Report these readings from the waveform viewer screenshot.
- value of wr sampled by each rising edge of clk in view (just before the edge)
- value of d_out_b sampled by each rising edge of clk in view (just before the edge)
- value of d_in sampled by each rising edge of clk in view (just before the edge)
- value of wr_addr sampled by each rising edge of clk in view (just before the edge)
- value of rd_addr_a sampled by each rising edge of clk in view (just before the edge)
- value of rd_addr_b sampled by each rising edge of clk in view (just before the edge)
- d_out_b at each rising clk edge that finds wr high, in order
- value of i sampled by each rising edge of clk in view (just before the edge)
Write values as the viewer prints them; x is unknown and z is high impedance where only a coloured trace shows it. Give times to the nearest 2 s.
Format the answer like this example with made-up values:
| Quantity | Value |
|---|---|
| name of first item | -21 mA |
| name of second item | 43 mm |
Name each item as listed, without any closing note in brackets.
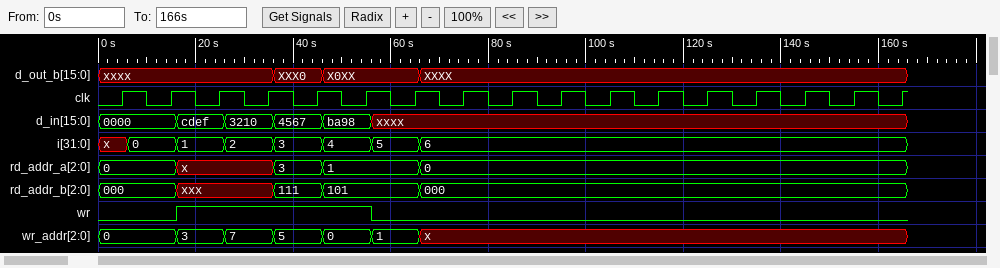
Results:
| Quantity | Value |
|---|---|
| value of wr sampled by each rising edge of clk in view | 0 0 1 1 1 1 0 0 0 0 0 0 0 0 0 0 0 |
| value of d_out_b sampled by each rising edge of clk in view | xxxx, xxxx, xxxx, xxxx, XXX0, X0XX, X0XX, XXXX, XXXX, XXXX, XXXX, XXXX, XXXX, XXXX, XXXX, XXXX, XXXX |
| value of d_in sampled by each rising edge of clk in view | 0000, 0000, cdef, 3210, 4567, ba98, xxxx, xxxx, xxxx, xxxx, xxxx, xxxx, xxxx, xxxx, xxxx, xxxx, xxxx |
| value of wr_addr sampled by each rising edge of clk in view | 0, 0, 3, 7, 5, 0, 1, x, x, x, x, x, x, x, x, x, x |
| value of rd_addr_a sampled by each rising edge of clk in view | 0, 0, x, x, 3, 1, 1, 0, 0, 0, 0, 0, 0, 0, 0, 0, 0 |
| value of rd_addr_b sampled by each rising edge of clk in view | 000, 000, xxx, xxx, 111, 101, 101, 000, 000, 000, 000, 000, 000, 000, 000, 000, 000 |
| d_out_b at each rising clk edge that finds wr high, in order | xxxx, xxxx, XXX0, X0XX |
| value of i sampled by each rising edge of clk in view | x, 0, 1, 2, 3, 4, 5, 6, 6, 6, 6, 6, 6, 6, 6, 6, 6 |
